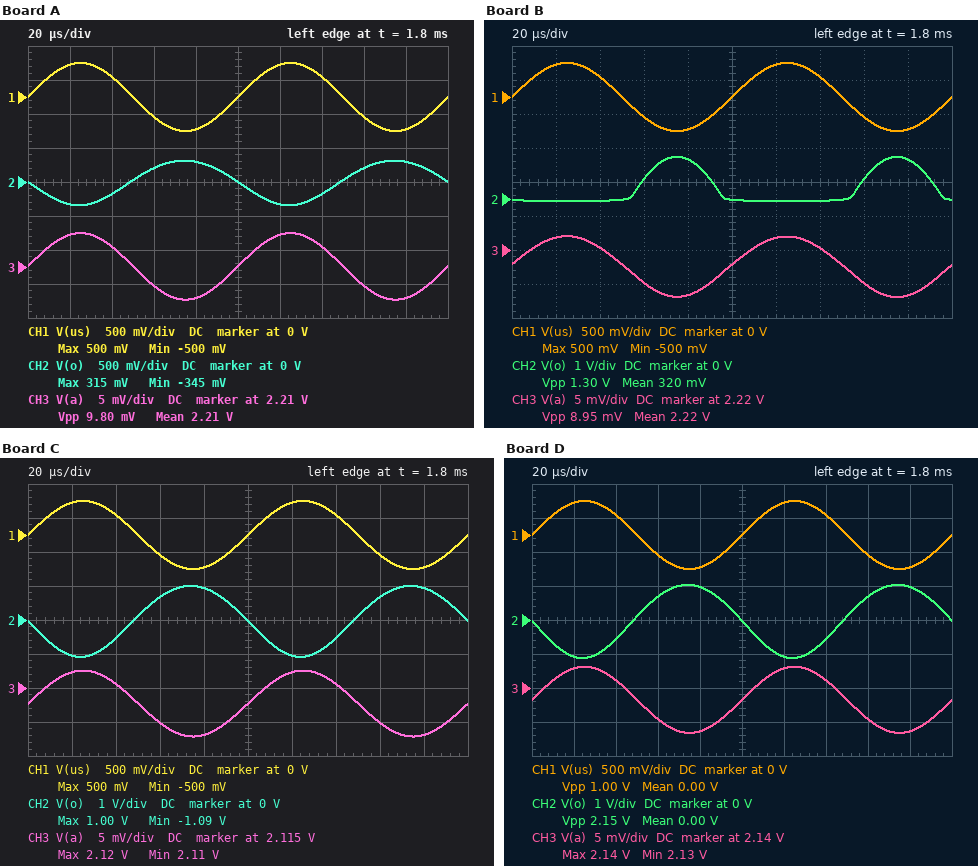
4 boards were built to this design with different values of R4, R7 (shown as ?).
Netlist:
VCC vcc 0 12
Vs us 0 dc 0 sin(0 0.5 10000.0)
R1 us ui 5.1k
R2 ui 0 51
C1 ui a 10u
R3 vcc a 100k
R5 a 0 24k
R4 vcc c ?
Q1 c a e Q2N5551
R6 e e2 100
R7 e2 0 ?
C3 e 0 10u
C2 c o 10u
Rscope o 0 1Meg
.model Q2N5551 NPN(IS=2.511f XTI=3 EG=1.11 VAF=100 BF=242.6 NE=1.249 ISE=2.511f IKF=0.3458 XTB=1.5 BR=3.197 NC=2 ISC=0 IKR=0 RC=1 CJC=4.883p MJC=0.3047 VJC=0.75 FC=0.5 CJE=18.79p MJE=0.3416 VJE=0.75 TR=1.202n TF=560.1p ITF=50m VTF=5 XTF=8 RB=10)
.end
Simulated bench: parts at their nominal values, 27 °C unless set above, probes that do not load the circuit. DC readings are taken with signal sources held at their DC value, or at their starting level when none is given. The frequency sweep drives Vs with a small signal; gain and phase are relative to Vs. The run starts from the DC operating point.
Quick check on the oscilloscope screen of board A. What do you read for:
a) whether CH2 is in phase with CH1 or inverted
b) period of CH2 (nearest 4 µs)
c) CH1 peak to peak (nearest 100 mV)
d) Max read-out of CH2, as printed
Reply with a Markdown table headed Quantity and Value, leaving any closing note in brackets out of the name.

| Quantity | Value |
|---|---|
| whether CH2 is in phase with CH1 or inverted | inverted |
| period of CH2 | 100 µs |
| CH1 peak to peak | 1.0 V |
| Max read-out of CH2, as printed | 315 mV |
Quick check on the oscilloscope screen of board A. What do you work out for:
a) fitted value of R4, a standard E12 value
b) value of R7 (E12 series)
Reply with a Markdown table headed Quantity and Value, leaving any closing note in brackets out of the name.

| Quantity | Value |
|---|---|
| fitted value of R4, a standard E12 value | 2.7 kΩ |
| value of R7 | 2.2 kΩ |
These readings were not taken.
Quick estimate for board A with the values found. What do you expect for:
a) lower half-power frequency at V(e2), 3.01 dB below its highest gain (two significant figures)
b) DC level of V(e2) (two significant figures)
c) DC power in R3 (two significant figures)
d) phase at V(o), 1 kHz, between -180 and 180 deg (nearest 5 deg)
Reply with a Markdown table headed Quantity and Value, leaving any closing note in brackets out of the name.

| Quantity | Value |
|---|---|
| lower half-power frequency at V(e2), 3.01 dB below its highest gain | 860 mHz |
| DC level of V(e2) | 1.5 V |
| DC power in R3 | 960 µW |
| phase at V(o), 1 kHz, between -180 and 180 deg | -160 deg |
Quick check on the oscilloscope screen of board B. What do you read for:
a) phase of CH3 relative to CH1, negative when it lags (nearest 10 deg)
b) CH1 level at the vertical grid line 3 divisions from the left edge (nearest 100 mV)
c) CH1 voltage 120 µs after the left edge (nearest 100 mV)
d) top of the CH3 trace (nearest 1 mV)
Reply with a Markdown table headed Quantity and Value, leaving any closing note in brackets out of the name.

| Quantity | Value |
|---|---|
| phase of CH3 relative to CH1, negative when it lags | 0 deg |
| CH1 level at the vertical grid line 3 divisions from the left edge | -300 mV |
| CH1 voltage 120 µs after the left edge | 500 mV |
| top of the CH3 trace | 2.222 V |
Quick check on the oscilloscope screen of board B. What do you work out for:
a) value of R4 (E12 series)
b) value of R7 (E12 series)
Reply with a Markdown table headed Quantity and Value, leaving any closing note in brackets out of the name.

| Quantity | Value |
|---|---|
| value of R4 | 27 kΩ |
| value of R7 | 3.9 kΩ |
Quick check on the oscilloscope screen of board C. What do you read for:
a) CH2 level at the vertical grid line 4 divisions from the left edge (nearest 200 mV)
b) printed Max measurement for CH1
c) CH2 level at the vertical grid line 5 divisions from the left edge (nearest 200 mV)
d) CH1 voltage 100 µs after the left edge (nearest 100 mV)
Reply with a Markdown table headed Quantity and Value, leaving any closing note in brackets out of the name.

| Quantity | Value |
|---|---|
| CH2 level at the vertical grid line 4 divisions from the left edge | 1.0 V |
| printed Max measurement for CH1 | 500 mV |
| CH2 level at the vertical grid line 5 divisions from the left edge | 0 V |
| CH1 voltage 100 µs after the left edge | 0 V |
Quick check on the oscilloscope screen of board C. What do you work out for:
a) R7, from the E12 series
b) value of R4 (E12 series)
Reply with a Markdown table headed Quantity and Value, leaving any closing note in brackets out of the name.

| Quantity | Value |
|---|---|
| R7, from the E12 series | 1 kΩ |
| value of R4 | 4.7 kΩ |
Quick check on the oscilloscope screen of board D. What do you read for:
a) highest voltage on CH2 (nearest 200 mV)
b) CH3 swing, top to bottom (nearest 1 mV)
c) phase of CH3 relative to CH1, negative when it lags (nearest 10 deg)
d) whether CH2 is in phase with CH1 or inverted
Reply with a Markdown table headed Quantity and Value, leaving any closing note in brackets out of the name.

| Quantity | Value |
|---|---|
| highest voltage on CH2 | 1.0 V |
| CH3 swing, top to bottom | 10 mV |
| phase of CH3 relative to CH1, negative when it lags | 0 deg |
| whether CH2 is in phase with CH1 or inverted | inverted |
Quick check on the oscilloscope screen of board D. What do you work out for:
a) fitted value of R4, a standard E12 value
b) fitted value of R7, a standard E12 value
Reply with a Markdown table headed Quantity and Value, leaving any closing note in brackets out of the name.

| Quantity | Value |
|---|---|
| fitted value of R4, a standard E12 value | 5.6 kΩ |
| fitted value of R7, a standard E12 value | 1.2 kΩ |
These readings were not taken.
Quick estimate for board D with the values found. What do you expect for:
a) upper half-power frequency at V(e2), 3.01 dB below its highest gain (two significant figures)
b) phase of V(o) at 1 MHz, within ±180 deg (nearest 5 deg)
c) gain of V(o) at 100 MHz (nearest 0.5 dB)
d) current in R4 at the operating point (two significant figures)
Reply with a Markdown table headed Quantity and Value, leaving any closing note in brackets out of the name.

| Quantity | Value |
|---|---|
| upper half-power frequency at V(e2), 3.01 dB below its highest gain | 650 Hz |
| phase of V(o) at 1 MHz, within ±180 deg | 160 deg |
| gain of V(o) at 100 MHz | -25.0 dB |
| current in R4 at the operating point | 1.1 mA |
